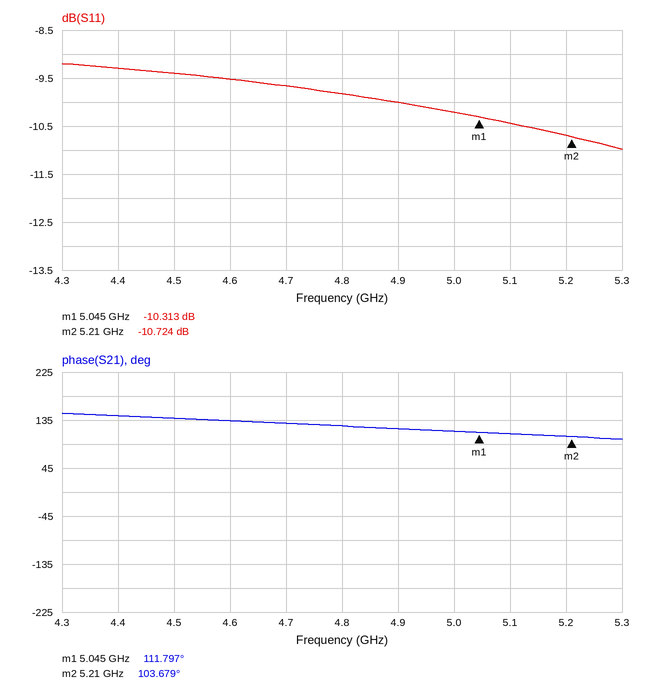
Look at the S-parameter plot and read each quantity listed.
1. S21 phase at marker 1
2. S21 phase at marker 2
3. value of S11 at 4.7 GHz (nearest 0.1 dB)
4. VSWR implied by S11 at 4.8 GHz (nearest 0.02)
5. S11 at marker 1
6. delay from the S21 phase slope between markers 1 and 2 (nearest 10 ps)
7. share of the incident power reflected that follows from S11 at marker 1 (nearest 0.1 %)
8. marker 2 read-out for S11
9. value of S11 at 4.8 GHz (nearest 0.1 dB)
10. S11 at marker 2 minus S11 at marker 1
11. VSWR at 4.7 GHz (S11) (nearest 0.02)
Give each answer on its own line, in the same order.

111.797°
103.679°
-9.7 dB
1.96
-10.313 dB
140 ps
9.3 %
-10.724 dB
-9.8 dB
-0.411 dB
1.98
